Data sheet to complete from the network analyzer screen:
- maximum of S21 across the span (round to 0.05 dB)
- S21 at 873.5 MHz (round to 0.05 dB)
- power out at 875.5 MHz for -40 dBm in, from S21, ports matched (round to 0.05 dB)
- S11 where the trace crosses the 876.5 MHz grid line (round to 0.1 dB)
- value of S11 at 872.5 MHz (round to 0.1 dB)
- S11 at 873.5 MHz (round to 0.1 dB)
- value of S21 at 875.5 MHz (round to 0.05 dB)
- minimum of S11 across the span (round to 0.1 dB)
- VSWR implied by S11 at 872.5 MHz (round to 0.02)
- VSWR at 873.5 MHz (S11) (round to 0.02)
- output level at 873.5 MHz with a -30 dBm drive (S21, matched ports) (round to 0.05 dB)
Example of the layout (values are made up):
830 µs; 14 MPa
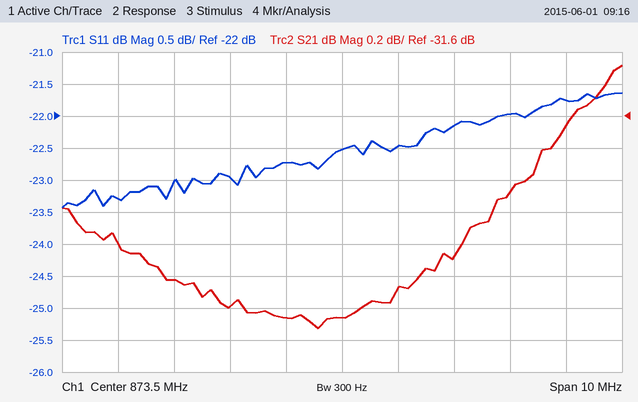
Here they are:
-31.30 dB; -32.85 dB; -72.50 dBm; -22.0 dB; -22.7 dB; -22.5 dB; -32.50 dB; -23.4 dB; 1.16; 1.16; -62.85 dBm
